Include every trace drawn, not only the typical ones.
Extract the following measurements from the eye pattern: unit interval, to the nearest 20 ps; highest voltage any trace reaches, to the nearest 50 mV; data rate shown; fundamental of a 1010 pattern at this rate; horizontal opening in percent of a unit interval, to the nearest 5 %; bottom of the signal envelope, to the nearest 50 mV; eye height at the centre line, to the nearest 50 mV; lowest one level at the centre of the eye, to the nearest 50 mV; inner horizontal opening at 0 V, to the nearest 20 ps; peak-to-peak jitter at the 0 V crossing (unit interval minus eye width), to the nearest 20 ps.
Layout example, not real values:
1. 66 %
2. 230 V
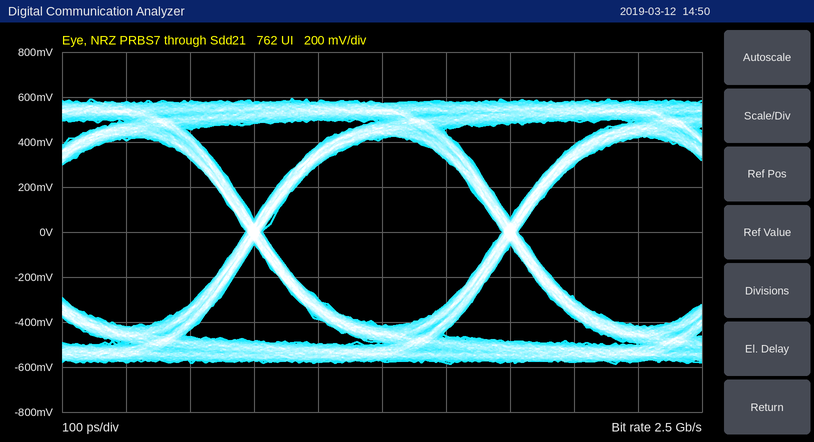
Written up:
1. 400 ps
2. 600 mV
3. 2.5 Gb/s
4. 1.25 GHz
5. 95 %
6. -600 mV
7. 850 mV
8. 400 mV
9. 380 ps
10. 20 ps
